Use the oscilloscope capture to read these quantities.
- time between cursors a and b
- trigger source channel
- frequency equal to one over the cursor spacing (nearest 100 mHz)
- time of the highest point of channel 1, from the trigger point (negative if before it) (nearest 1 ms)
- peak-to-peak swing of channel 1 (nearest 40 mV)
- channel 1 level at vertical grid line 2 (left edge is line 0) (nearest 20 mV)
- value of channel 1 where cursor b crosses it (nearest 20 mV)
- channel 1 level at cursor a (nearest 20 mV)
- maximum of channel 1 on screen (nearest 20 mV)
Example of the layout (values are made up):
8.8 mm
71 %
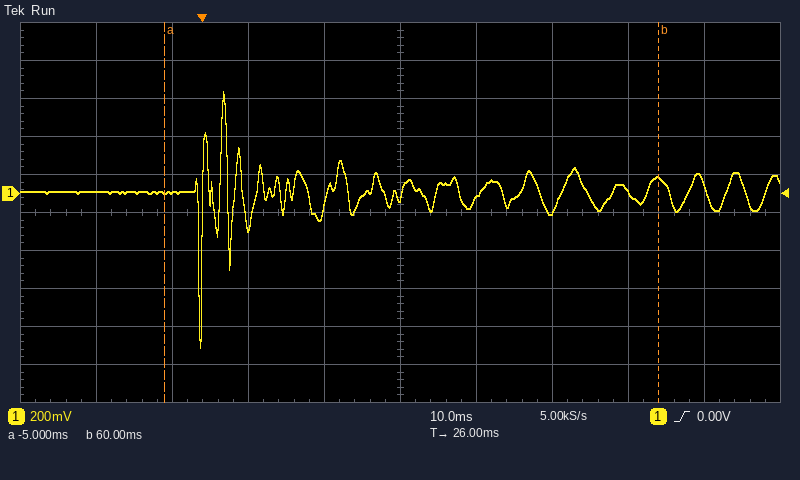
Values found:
65 ms
channel 1
15.4 Hz
+3 ms
1.36 V
0 mV
80 mV
0 mV
540 mV
